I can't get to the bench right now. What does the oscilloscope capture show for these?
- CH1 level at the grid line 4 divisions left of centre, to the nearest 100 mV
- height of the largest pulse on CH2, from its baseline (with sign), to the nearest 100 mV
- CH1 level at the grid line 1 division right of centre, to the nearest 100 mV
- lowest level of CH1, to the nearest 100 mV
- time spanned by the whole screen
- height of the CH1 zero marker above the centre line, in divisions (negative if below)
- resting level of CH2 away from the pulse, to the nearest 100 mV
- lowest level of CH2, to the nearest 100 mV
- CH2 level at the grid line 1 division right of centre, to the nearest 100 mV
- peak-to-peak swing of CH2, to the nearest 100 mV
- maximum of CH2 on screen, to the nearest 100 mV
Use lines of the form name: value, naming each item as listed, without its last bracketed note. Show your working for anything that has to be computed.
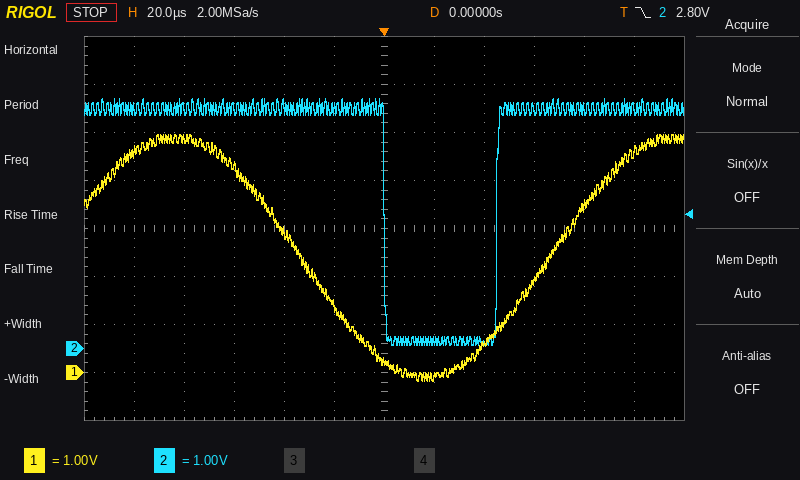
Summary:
CH1 level at the grid line 4 divisions left of centre, to the nearest 100 mV: 4.9 V
height of the largest pulse on CH2, from its baseline (with sign), to the nearest 100 mV: 100 mV − (5.0 V) = -4.9 V
CH1 level at the grid line 1 division right of centre, to the nearest 100 mV: -100 mV
lowest level of CH1, to the nearest 100 mV: -200 mV
time spanned by the whole screen: 240 µs
height of the CH1 zero marker above the centre line, in divisions: -3.0 div
resting level of CH2 away from the pulse, to the nearest 100 mV: 5.0 V
lowest level of CH2, to the nearest 100 mV: 100 mV
CH2 level at the grid line 1 division right of centre, to the nearest 100 mV: 200 mV
peak-to-peak swing of CH2, to the nearest 100 mV: 5.2 V − (100 mV) = 5.1 V
maximum of CH2 on screen, to the nearest 100 mV: 5.2 V
